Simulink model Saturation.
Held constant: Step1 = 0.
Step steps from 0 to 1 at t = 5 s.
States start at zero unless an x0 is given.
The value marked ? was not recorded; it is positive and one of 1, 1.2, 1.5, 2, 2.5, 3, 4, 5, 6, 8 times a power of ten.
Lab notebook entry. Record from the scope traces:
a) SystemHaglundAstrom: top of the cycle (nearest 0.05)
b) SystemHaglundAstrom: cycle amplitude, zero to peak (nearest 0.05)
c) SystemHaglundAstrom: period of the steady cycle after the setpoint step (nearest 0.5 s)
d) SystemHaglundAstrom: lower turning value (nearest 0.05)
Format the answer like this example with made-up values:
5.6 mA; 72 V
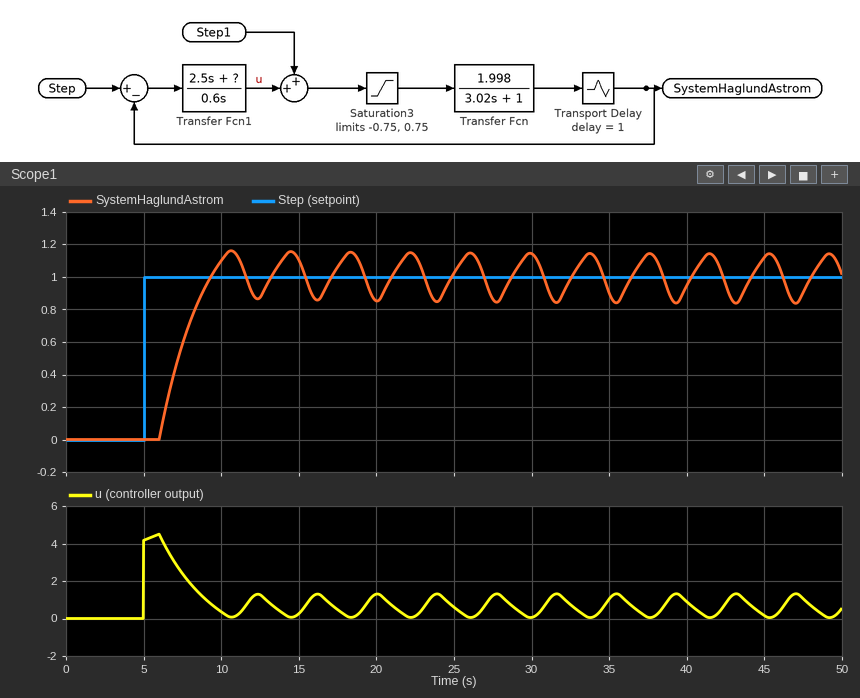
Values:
1.15; 0.15; 4.0 s; 0.85
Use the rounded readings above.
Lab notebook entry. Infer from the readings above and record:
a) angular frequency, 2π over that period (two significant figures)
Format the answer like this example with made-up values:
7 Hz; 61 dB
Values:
1.6 rad/s
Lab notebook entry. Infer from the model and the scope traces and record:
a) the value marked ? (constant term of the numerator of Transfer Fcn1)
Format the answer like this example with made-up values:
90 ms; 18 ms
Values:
0.2
